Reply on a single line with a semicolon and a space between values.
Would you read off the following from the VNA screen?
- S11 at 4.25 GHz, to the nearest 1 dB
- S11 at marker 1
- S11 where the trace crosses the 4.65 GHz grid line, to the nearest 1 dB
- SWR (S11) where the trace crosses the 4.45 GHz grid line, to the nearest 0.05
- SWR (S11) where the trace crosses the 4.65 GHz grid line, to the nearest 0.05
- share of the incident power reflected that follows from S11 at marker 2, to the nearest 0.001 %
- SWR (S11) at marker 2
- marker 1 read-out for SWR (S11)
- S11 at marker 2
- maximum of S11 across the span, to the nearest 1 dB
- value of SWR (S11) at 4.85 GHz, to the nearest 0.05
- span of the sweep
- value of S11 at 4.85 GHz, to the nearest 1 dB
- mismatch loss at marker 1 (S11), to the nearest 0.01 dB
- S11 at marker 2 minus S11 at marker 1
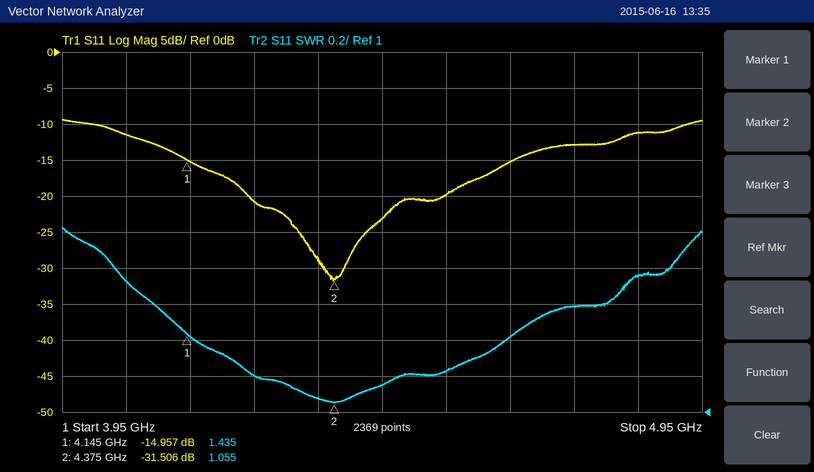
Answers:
-21 dB; -14.957 dB; -15 dB; 1.15; 1.40; 0.071 %; 1.055; 1.435; -31.506 dB; -9 dB; 1.75; 1 GHz; -11 dB; 0.14 dB; -16.549 dB
